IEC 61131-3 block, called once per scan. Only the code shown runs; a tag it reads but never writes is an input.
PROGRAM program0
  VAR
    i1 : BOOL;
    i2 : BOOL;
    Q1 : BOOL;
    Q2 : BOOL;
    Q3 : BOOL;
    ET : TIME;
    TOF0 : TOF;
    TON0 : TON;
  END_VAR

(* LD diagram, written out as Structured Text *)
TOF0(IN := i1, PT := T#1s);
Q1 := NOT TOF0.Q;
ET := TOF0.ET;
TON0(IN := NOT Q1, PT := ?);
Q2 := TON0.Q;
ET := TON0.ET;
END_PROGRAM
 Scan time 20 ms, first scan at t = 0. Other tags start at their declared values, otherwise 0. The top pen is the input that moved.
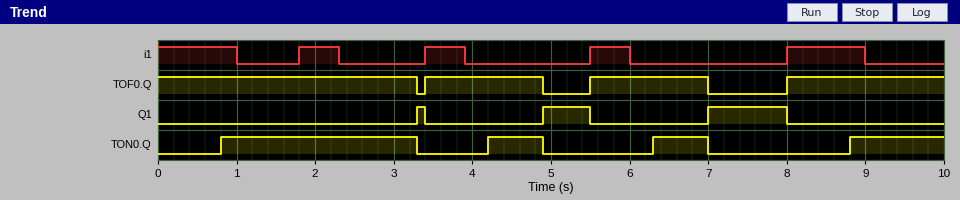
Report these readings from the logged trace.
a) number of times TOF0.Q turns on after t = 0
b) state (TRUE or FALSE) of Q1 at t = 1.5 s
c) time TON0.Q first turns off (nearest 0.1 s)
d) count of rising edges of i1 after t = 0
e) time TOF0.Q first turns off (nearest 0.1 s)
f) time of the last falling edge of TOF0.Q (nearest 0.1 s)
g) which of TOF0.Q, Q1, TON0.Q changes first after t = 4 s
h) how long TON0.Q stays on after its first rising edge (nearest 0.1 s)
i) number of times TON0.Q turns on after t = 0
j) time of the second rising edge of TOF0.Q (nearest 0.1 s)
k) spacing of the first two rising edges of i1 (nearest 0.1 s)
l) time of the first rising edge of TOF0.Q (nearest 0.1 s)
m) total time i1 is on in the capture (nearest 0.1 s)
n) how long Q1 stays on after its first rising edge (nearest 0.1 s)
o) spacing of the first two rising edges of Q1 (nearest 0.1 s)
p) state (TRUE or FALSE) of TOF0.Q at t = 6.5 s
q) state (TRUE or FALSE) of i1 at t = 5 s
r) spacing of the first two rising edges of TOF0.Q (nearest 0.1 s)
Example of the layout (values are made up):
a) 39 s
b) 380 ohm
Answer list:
a) 3
b) FALSE
c) 3.3 s
d) 4
e) 3.3 s
f) 7.0 s
g) TON0.Q
h) 2.5 s
i) 4
j) 5.5 s
k) 1.6 s
l) 3.4 s
m) 3.5 s
n) 0.1 s
o) 1.6 s
p) TRUE
q) FALSE
r) 2.1 s
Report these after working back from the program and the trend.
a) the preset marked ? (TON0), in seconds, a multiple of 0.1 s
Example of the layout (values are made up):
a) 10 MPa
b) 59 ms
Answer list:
a) 0.8 s
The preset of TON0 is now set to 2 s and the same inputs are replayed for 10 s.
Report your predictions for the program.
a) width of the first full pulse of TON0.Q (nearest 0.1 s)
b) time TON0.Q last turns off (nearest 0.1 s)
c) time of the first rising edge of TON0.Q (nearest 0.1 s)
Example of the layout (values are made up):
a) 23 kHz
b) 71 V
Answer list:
a) 1.3 s
b) 3.3 s
c) 2.0 s
